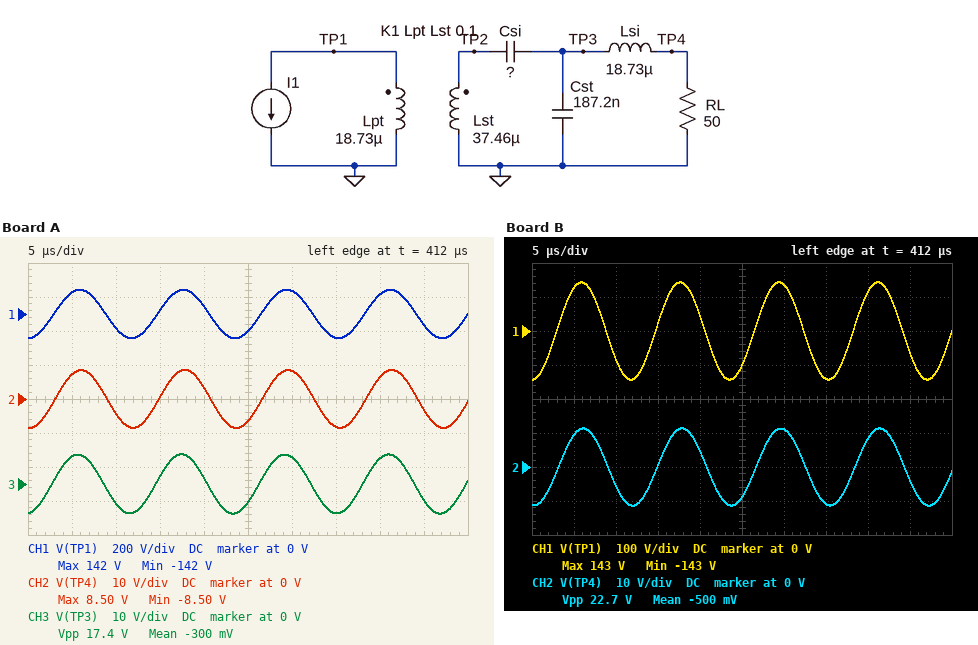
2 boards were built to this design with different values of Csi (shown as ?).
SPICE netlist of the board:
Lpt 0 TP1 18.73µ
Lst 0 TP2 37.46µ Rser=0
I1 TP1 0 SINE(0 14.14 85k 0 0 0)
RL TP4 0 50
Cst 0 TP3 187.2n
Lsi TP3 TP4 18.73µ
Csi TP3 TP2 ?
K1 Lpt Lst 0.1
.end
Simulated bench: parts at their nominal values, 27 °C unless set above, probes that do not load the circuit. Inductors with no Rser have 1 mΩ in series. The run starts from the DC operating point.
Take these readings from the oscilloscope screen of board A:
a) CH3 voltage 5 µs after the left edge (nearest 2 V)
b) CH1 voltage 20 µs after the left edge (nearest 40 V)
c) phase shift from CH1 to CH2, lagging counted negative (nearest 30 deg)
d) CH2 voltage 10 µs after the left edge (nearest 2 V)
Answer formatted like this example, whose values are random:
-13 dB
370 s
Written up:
8 V
40 V
0 deg
-4 V
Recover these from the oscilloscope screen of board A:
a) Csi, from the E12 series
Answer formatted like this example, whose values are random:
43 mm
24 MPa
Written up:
56 nF
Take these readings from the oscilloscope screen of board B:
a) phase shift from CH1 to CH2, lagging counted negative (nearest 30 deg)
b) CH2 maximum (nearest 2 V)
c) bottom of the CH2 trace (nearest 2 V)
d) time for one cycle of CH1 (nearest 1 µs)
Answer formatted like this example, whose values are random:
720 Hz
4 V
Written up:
0 deg
12 V
-12 V
12 µs
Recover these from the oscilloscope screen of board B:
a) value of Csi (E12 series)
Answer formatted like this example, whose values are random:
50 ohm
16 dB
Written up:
68 nF
